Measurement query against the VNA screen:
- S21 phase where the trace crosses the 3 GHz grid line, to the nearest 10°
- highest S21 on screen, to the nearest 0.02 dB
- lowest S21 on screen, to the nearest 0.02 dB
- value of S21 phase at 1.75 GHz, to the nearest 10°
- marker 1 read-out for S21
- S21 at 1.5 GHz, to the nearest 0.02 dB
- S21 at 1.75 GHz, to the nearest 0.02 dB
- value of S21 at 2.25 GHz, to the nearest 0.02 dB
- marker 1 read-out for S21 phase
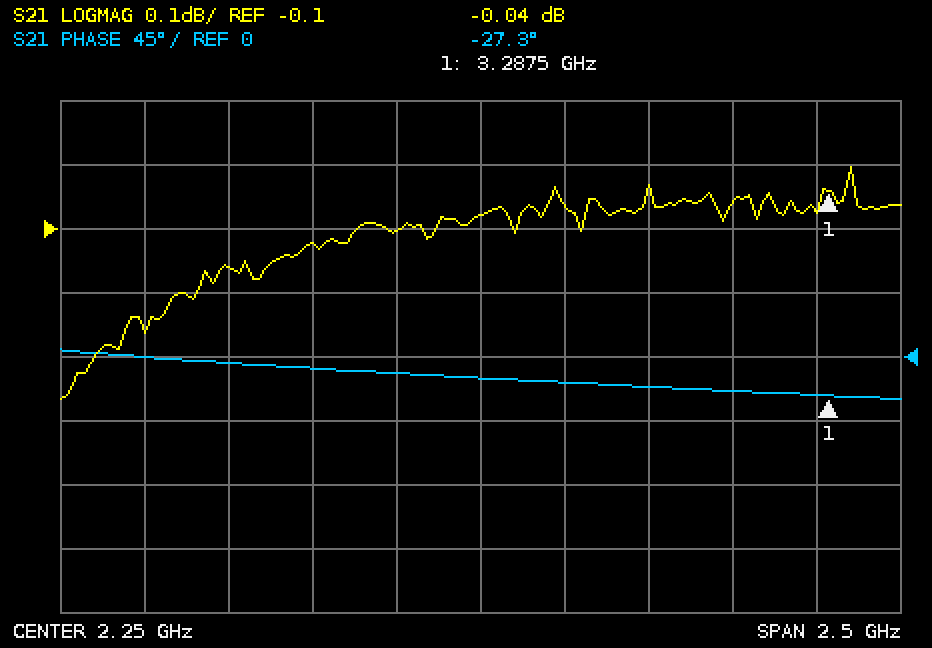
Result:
-20°
0.00 dB
-0.36 dB
-10°
-0.04 dB
-0.16 dB
-0.12 dB
-0.08 dB
-27.3°
